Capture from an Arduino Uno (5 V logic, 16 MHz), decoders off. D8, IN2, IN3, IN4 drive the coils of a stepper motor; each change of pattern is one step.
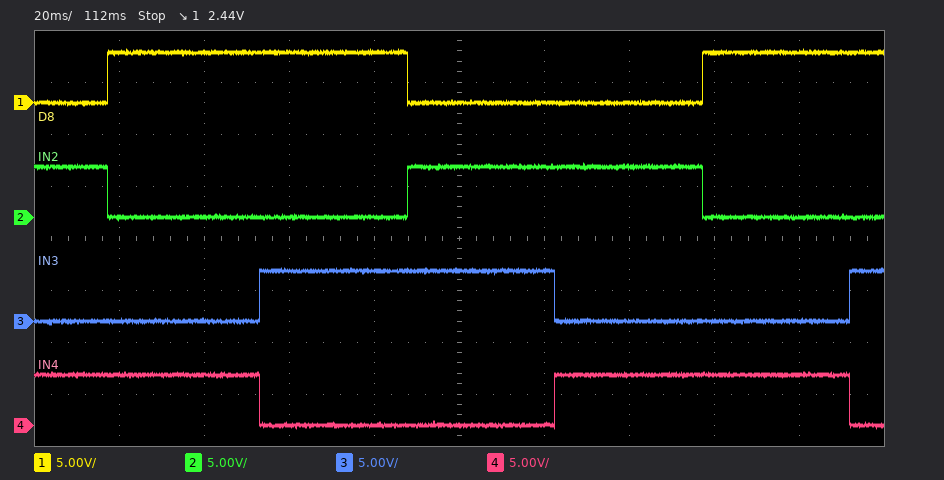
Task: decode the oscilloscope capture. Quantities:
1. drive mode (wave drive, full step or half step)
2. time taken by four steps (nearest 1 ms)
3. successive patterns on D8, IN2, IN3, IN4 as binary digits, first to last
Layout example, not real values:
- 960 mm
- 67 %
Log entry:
- full step
- 140 ms
- 0101 1001 1010 0110 0101 1001 1010
